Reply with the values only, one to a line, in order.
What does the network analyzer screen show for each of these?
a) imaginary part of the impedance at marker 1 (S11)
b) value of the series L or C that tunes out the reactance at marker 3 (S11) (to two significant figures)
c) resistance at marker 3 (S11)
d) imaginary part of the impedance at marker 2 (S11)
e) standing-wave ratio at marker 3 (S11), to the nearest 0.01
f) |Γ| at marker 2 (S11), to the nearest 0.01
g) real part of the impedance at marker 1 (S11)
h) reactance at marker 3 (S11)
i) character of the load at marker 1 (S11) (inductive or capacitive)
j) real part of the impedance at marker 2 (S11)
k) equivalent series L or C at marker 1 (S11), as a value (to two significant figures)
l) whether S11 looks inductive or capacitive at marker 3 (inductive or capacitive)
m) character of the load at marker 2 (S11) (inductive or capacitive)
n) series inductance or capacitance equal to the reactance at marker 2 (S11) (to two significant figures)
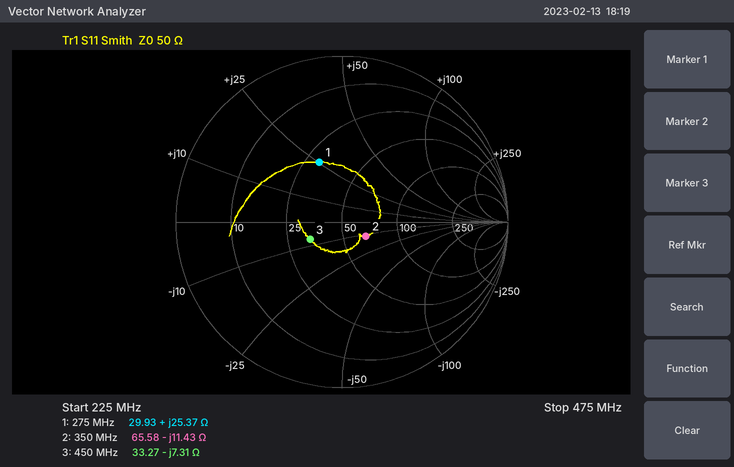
+25.37 Ω
2.6 nH
33.27 Ω
-11.43 Ω
1.56
0.17
29.93 Ω
-7.31 Ω
inductive
65.58 Ω
15 nH
capacitive
capacitive
40 pF
